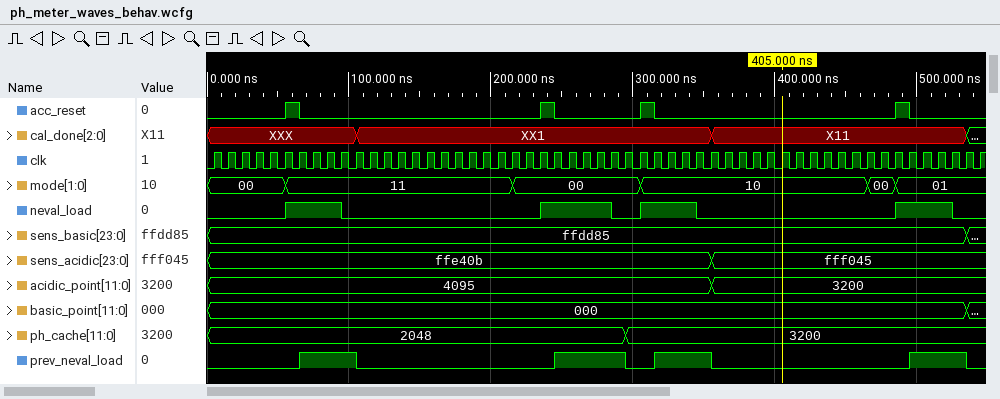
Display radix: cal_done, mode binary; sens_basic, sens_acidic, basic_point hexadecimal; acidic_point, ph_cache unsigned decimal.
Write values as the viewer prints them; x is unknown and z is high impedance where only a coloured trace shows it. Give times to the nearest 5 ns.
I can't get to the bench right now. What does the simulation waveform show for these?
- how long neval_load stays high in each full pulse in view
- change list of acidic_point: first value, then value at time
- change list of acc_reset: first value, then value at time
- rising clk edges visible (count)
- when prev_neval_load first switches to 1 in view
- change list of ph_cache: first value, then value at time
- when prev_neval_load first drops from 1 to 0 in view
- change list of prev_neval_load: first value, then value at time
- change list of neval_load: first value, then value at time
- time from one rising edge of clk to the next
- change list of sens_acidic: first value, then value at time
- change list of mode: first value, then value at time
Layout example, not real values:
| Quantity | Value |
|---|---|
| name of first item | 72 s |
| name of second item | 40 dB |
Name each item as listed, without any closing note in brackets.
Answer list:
| Quantity | Value |
|---|---|
| how long neval_load stays high in each full pulse in view | 40 ns, 50 ns, 40 ns, 40 ns |
| change list of acidic_point: first value, then value at time | 4095, 3200 at 355 ns |
| change list of acc_reset: first value, then value at time | 0, 1 at 55 ns, 0 at 65 ns, 1 at 235 ns, 0 at 245 ns, 1 at 305 ns, 0 at 315 ns, 1 at 485 ns, 0 at 495 ns |
| rising clk edges visible | 55 |
| when prev_neval_load first switches to 1 in view | 65 ns |
| change list of ph_cache: first value, then value at time | 2048, 3200 at 295 ns |
| when prev_neval_load first drops from 1 to 0 in view | 105 ns |
| change list of prev_neval_load: first value, then value at time | 0, 1 at 65 ns, 0 at 105 ns, 1 at 245 ns, 0 at 295 ns, 1 at 315 ns, 0 at 355 ns, 1 at 495 ns, 0 at 535 ns |
| change list of neval_load: first value, then value at time | 0, 1 at 55 ns, 0 at 95 ns, 1 at 235 ns, 0 at 285 ns, 1 at 305 ns, 0 at 345 ns, 1 at 485 ns, 0 at 525 ns |
| time from one rising edge of clk to the next | 10 ns |
| change list of sens_acidic: first value, then value at time | ffe40b, fff045 at 355 ns |
| change list of mode: first value, then value at time | 00, 11 at 55 ns, 00 at 215 ns, 10 at 305 ns, 00 at 465 ns, 01 at 485 ns |
